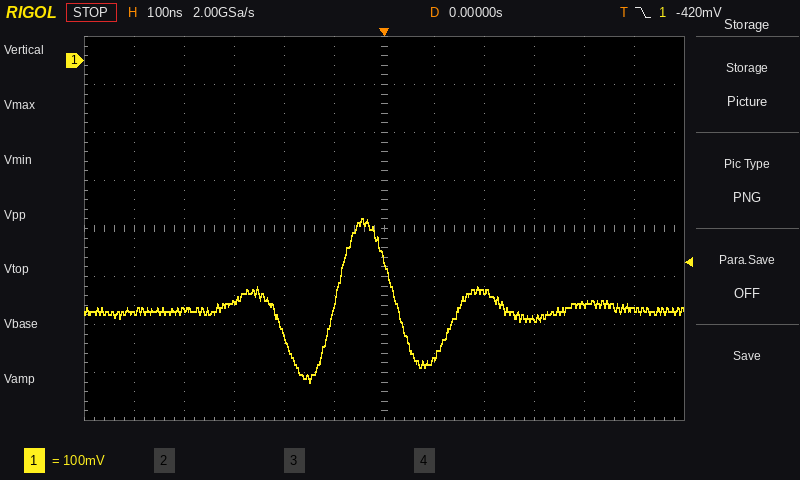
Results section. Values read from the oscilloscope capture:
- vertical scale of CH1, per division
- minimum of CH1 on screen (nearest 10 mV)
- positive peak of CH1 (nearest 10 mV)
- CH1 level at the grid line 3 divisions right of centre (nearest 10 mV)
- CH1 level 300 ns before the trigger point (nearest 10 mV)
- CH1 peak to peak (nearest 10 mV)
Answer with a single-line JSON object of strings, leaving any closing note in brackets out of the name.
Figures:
{"vertical scale of CH1, per division": "100 mV", "minimum of CH1 on screen": "-670 mV", "positive peak of CH1": "-330 mV", "CH1 level at the grid line 3 divisions right of centre": "-540 mV", "CH1 level 300 ns before the trigger point": "-500 mV", "CH1 peak to peak": "340 mV"}
